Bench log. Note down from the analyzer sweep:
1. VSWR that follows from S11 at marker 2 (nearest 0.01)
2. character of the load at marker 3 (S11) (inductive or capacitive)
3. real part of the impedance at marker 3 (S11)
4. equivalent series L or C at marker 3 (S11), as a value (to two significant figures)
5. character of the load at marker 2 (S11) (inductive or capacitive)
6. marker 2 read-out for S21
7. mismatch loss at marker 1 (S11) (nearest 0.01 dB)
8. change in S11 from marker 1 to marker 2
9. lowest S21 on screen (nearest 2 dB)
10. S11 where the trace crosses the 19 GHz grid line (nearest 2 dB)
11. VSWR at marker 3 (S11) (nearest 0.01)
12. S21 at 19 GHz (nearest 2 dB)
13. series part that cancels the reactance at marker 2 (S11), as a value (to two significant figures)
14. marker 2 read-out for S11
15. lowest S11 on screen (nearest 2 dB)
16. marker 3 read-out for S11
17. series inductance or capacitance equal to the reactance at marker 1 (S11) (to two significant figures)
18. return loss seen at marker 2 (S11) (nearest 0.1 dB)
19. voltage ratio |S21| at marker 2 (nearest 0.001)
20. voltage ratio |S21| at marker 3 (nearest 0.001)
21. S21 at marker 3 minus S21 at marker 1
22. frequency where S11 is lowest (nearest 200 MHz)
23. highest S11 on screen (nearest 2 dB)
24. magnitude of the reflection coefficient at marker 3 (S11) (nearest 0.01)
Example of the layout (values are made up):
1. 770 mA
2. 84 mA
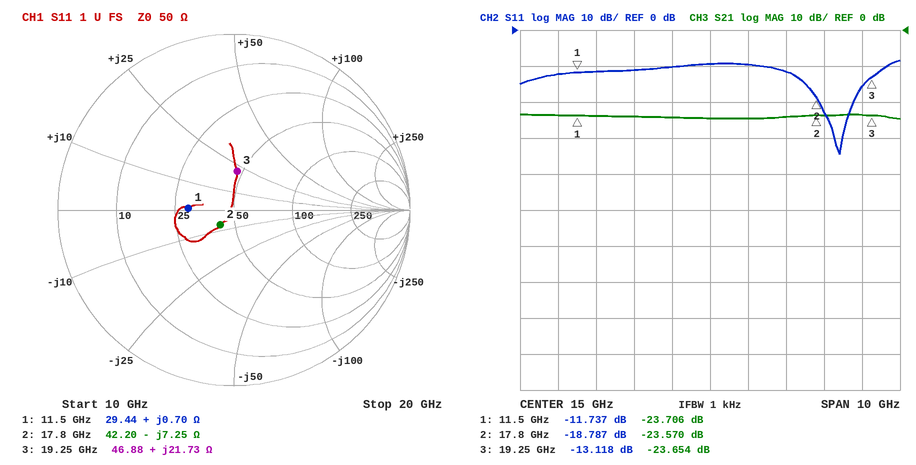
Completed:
1. 1.26
2. inductive
3. 46.88 Ω
4. 180 pH
5. capacitive
6. -23.570 dB
7. 0.30 dB
8. -7.050 dB
9. -24 dB
10. -16 dB
11. 1.57
12. -24 dB
13. 65 pH
14. -18.787 dB
15. -34 dB
16. -13.118 dB
17. 9.7 pH
18. 18.8 dB
19. 0.066
20. 0.066
21. 0.052 dB
22. 18.4 GHz
23. -8 dB
24. 0.22
